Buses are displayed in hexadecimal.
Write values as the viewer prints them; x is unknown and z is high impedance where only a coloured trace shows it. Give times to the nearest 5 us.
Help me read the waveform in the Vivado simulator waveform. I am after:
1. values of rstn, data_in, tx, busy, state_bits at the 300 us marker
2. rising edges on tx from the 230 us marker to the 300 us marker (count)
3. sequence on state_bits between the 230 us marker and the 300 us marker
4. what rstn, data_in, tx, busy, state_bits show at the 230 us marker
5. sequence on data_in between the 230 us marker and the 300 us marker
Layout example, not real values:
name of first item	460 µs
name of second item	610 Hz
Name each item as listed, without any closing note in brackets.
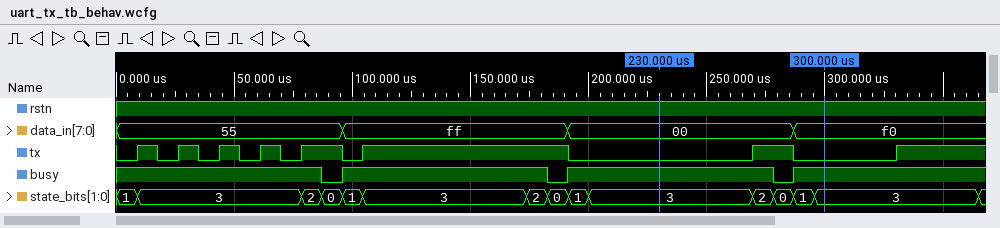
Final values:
values of rstn, data_in, tx, busy, state_bits at the 300 us marker	rstn=1, data_in=f0, tx=0, busy=1, state_bits=3
rising edges on tx from the 230 us marker to the 300 us marker	1
sequence on state_bits between the 230 us marker and the 300 us marker	3, 2, 0, 1, 3
what rstn, data_in, tx, busy, state_bits show at the 230 us marker	rstn=1, data_in=00, tx=0, busy=1, state_bits=3
sequence on data_in between the 230 us marker and the 300 us marker	00, f0
